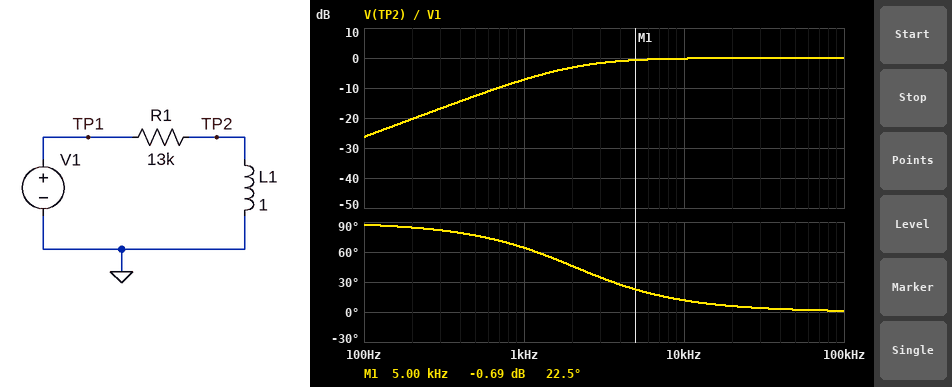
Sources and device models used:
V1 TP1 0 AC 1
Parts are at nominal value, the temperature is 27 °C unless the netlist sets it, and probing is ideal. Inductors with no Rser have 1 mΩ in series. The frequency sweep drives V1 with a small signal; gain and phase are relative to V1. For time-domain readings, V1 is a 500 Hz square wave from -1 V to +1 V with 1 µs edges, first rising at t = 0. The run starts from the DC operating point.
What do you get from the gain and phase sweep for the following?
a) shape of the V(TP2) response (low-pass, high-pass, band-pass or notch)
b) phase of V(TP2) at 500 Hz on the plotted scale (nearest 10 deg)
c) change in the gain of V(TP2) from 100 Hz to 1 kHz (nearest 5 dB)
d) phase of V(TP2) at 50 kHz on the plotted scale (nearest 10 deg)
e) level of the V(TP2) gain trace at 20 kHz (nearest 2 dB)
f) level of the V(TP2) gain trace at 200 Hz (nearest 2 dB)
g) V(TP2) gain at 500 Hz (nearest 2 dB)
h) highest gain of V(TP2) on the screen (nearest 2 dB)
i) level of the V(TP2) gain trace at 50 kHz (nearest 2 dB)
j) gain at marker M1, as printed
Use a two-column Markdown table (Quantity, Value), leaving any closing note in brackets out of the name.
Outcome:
| Quantity | Value |
|---|---|
| shape of the V(TP2) response | high-pass |
| phase of V(TP2) at 500 Hz on the plotted scale | 80 deg |
| change in the gain of V(TP2) from 100 Hz to 1 kHz | 20 dB |
| phase of V(TP2) at 50 kHz on the plotted scale | 0 deg |
| level of the V(TP2) gain trace at 20 kHz | 0 dB |
| level of the V(TP2) gain trace at 200 Hz | -20 dB |
| V(TP2) gain at 500 Hz | -12 dB |
| highest gain of V(TP2) on the screen | 0 dB |
| level of the V(TP2) gain trace at 50 kHz | 0 dB |
| gain at marker M1, as printed | -0.69 dB |
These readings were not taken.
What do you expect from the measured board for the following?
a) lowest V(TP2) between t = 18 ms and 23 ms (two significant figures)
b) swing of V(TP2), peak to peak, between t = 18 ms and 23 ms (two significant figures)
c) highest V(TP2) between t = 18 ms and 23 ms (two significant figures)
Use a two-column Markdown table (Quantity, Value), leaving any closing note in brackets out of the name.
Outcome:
| Quantity | Value |
|---|---|
| lowest V(TP2) between t = 18 ms and 23 ms | -2.0 V |
| swing of V(TP2), peak to peak, between t = 18 ms and 23 ms | 4.0 V |
| highest V(TP2) between t = 18 ms and 23 ms | 2.0 V |
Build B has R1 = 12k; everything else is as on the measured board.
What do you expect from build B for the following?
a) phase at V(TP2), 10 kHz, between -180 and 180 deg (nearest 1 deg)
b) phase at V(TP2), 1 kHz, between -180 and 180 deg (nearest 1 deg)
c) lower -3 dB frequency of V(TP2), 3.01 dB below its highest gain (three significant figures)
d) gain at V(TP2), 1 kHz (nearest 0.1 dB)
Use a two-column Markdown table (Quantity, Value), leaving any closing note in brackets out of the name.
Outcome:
| Quantity | Value |
|---|---|
| phase at V(TP2), 10 kHz, between -180 and 180 deg | 11 deg |
| phase at V(TP2), 1 kHz, between -180 and 180 deg | 62 deg |
| lower -3 dB frequency of V(TP2), 3.01 dB below its highest gain | 1.91 kHz |
| gain at V(TP2), 1 kHz | -6.7 dB |
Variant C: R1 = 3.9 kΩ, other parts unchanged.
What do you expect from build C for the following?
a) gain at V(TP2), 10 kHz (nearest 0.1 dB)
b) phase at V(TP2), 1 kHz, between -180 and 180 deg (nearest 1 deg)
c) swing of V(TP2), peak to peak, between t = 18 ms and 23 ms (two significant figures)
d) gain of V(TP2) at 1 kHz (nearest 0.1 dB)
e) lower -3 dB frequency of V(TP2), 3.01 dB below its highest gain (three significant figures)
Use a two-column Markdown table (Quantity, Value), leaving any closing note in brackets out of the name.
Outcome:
| Quantity | Value |
|---|---|
| gain at V(TP2), 10 kHz | 0 dB |
| phase at V(TP2), 1 kHz, between -180 and 180 deg | 32 deg |
| swing of V(TP2), peak to peak, between t = 18 ms and 23 ms | 3.9 V |
| gain of V(TP2) at 1 kHz | -1.4 dB |
| lower -3 dB frequency of V(TP2), 3.01 dB below its highest gain | 621 Hz |
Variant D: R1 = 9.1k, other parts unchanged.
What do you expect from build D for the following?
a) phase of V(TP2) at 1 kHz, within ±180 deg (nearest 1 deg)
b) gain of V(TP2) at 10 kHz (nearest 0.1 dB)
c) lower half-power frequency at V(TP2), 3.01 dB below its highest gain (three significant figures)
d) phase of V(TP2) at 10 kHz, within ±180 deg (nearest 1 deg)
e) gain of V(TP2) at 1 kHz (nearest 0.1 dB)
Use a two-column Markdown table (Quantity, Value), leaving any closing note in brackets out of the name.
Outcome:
| Quantity | Value |
|---|---|
| phase of V(TP2) at 1 kHz, within ±180 deg | 55 deg |
| gain of V(TP2) at 10 kHz | -0.1 dB |
| lower half-power frequency at V(TP2), 3.01 dB below its highest gain | 1.45 kHz |
| phase of V(TP2) at 10 kHz, within ±180 deg | 8 deg |
| gain of V(TP2) at 1 kHz | -4.9 dB |
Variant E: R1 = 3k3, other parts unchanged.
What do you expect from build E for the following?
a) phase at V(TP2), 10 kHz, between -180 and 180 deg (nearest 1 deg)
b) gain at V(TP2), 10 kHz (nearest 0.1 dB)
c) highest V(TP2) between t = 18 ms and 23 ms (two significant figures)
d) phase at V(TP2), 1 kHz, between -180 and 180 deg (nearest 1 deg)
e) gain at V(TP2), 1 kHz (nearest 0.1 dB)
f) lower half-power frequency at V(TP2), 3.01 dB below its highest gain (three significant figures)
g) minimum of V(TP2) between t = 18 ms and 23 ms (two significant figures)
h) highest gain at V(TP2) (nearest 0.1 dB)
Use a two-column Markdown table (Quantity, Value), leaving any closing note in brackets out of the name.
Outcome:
| Quantity | Value |
|---|---|
| phase at V(TP2), 10 kHz, between -180 and 180 deg | 3 deg |
| gain at V(TP2), 10 kHz | 0 dB |
| highest V(TP2) between t = 18 ms and 23 ms | 1.9 V |
| phase at V(TP2), 1 kHz, between -180 and 180 deg | 28 deg |
| gain at V(TP2), 1 kHz | -1.1 dB |
| lower half-power frequency at V(TP2), 3.01 dB below its highest gain | 525 Hz |
| minimum of V(TP2) between t = 18 ms and 23 ms | -1.9 V |
| highest gain at V(TP2) | 0 dB |
